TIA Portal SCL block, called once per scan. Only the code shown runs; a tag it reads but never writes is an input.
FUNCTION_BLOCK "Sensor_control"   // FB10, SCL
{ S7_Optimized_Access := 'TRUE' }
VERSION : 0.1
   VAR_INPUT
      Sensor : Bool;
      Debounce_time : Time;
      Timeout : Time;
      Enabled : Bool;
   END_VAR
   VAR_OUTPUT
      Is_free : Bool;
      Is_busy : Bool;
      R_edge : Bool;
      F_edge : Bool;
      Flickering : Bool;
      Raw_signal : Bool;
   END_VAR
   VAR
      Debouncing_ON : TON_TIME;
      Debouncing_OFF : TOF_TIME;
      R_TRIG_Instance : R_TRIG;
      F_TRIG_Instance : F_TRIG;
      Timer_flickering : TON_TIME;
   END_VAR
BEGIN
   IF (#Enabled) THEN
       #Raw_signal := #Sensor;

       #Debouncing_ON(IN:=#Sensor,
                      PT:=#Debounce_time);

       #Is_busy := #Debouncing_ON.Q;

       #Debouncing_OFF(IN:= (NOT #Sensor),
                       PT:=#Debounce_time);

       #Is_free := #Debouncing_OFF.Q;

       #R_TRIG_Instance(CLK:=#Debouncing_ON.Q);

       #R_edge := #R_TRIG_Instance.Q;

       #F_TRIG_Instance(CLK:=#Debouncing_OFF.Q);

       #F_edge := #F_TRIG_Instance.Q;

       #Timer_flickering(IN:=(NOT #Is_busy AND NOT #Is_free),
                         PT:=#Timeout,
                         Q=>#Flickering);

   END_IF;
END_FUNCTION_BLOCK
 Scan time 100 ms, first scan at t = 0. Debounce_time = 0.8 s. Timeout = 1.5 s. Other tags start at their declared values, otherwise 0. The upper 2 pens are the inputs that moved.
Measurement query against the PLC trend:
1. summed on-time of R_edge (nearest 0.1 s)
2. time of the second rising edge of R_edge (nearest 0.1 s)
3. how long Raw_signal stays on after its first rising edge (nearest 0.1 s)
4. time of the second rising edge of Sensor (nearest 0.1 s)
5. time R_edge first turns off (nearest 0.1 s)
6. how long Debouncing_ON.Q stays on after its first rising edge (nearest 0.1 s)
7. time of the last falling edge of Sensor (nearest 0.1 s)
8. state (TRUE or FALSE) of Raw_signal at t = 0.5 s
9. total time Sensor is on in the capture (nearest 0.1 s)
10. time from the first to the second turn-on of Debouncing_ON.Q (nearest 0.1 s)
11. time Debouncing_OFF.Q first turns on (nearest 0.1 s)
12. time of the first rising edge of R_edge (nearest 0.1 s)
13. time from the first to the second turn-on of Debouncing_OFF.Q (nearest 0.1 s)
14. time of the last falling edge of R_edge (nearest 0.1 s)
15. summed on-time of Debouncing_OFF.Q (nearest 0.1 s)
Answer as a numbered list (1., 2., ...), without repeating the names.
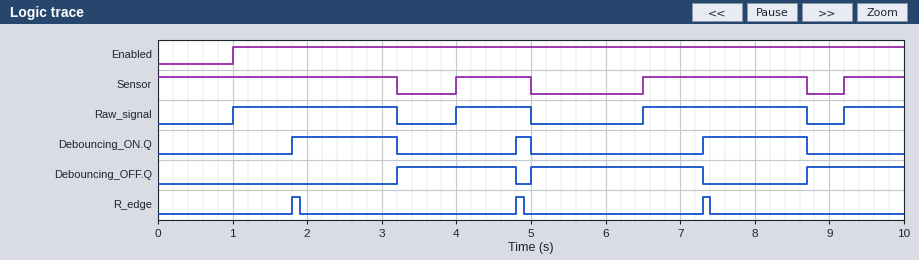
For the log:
1. 0.3 s
2. 4.8 s
3. 2.2 s
4. 6.5 s
5. 1.9 s
6. 1.4 s
7. 8.7 s
8. FALSE
9. 7.2 s
10. 3.0 s
11. 3.2 s
12. 1.8 s
13. 1.8 s
14. 7.4 s
15. 5.2 s
